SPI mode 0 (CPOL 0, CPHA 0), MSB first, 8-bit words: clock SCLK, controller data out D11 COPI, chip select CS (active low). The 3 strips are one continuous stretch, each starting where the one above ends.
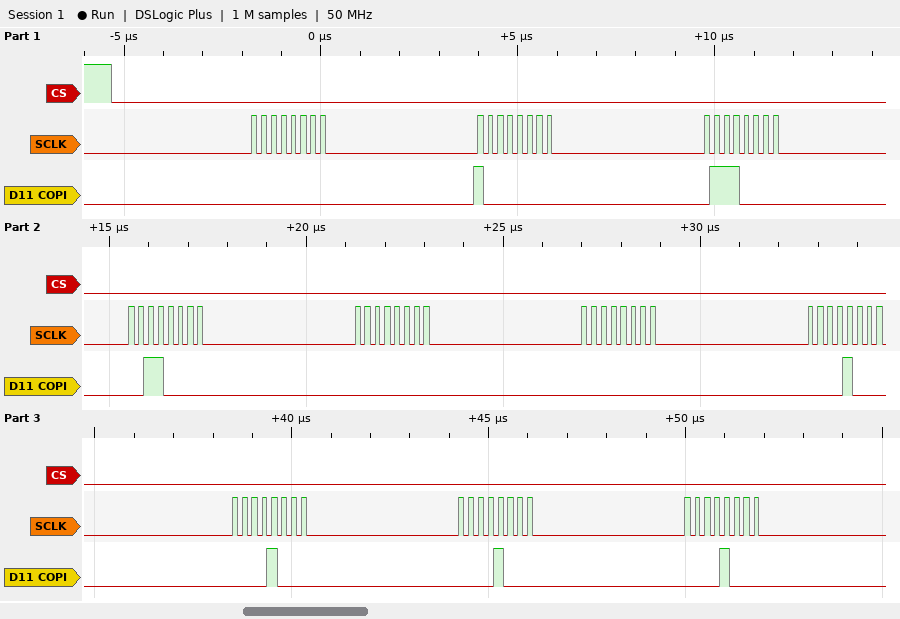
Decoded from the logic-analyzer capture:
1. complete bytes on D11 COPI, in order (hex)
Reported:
00 80 70 30 00 00 08 08 08 08
